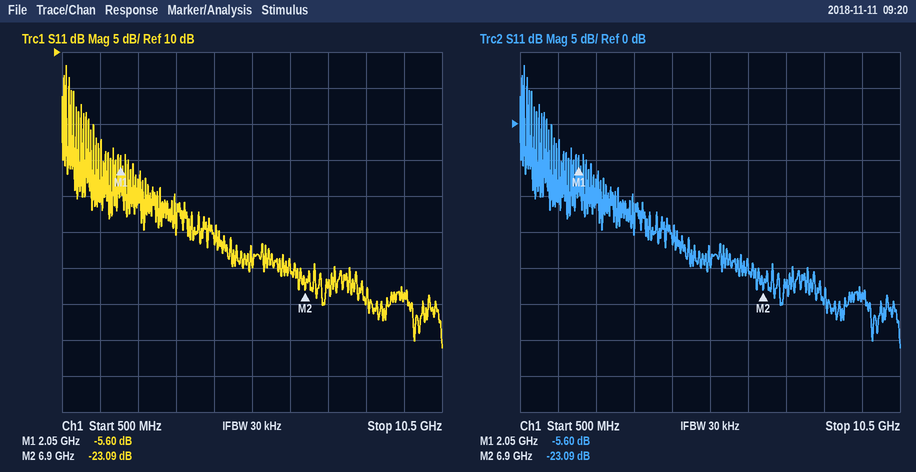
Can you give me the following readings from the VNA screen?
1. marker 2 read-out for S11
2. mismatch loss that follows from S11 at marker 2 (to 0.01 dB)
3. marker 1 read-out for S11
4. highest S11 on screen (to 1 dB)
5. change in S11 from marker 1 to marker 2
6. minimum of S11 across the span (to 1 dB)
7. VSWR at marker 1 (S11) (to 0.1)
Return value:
-23.09 dB
0.02 dB
-5.60 dB
8 dB
-17.49 dB
-31 dB
3.2
